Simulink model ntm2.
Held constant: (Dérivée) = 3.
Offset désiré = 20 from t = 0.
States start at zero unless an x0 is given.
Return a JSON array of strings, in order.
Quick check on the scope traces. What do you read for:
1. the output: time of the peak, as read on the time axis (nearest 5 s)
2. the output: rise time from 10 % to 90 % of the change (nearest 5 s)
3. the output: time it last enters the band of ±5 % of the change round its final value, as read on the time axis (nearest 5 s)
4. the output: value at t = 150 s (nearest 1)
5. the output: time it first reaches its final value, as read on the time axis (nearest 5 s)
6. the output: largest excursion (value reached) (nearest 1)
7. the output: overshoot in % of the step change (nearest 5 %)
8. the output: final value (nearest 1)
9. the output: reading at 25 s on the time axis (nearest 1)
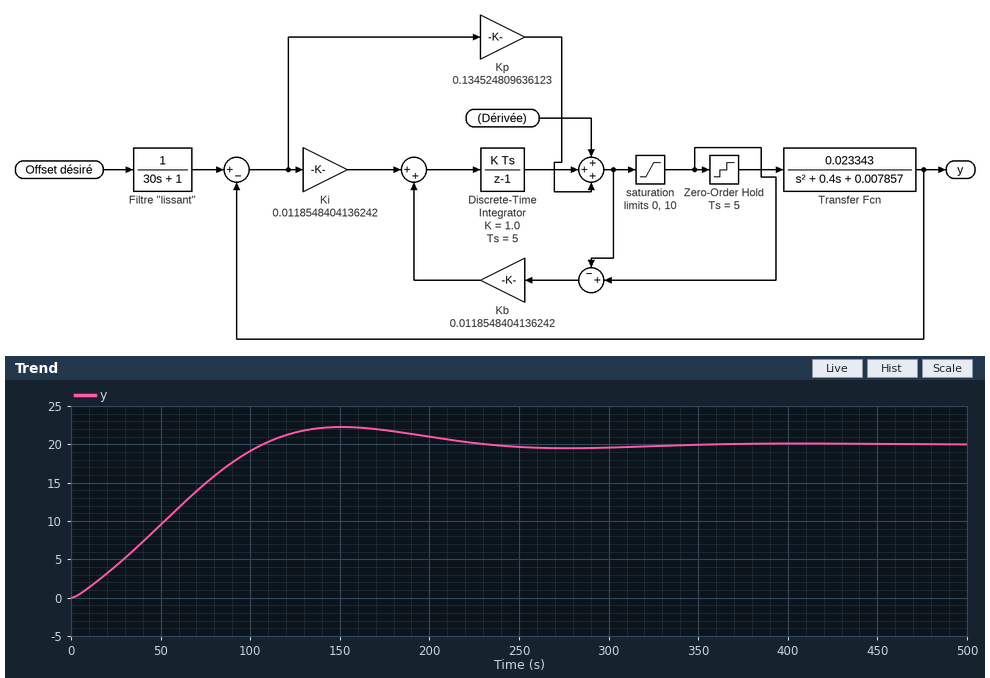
["150 s", "80 s", "200 s", "22", "105 s", "22", "10 %", "20", "4"]
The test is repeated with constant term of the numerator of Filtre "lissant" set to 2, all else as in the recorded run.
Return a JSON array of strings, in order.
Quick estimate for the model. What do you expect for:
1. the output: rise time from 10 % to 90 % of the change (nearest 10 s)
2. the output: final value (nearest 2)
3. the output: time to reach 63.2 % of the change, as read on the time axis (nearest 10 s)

["110 s", "30", "70 s"]
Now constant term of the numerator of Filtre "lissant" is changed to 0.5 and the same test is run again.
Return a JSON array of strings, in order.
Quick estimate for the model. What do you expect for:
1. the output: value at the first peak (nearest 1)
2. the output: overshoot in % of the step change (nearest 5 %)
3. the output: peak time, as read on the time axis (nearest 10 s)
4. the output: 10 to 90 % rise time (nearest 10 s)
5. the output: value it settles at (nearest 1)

["11", "10 %", "130 s", "70 s", "10"]
